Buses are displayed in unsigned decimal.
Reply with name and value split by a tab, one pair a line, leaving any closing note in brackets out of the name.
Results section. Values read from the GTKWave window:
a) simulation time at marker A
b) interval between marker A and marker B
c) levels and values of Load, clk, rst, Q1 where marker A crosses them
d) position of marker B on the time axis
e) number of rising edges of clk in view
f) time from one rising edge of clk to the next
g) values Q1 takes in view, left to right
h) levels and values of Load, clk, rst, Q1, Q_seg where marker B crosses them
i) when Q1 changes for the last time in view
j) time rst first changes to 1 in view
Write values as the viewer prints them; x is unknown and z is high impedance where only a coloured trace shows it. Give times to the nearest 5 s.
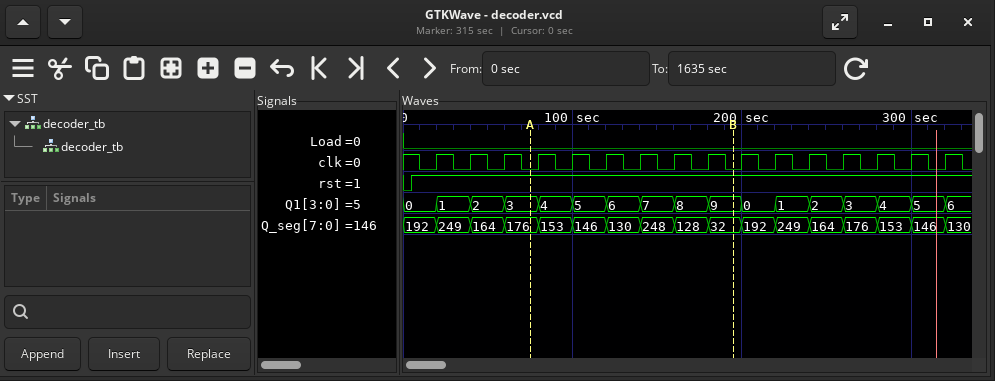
simulation time at marker A	75 s
interval between marker A and marker B	120 s
levels and values of Load, clk, rst, Q1 where marker A crosses them	Load=0, clk=0, rst=1, Q1=3
position of marker B on the time axis	195 s
number of rising edges of clk in view	16
time from one rising edge of clk to the next	20 s
values Q1 takes in view, left to right	0, 1, 2, 3, 4, 5, 6, 7, 8, 9, 0, 1, 2, 3, 4, 5, 6
levels and values of Load, clk, rst, Q1, Q_seg where marker B crosses them	Load=0, clk=0, rst=1, Q1=9, Q_seg=32
when Q1 changes for the last time in view	320 s
time rst first changes to 1 in view	5 s
